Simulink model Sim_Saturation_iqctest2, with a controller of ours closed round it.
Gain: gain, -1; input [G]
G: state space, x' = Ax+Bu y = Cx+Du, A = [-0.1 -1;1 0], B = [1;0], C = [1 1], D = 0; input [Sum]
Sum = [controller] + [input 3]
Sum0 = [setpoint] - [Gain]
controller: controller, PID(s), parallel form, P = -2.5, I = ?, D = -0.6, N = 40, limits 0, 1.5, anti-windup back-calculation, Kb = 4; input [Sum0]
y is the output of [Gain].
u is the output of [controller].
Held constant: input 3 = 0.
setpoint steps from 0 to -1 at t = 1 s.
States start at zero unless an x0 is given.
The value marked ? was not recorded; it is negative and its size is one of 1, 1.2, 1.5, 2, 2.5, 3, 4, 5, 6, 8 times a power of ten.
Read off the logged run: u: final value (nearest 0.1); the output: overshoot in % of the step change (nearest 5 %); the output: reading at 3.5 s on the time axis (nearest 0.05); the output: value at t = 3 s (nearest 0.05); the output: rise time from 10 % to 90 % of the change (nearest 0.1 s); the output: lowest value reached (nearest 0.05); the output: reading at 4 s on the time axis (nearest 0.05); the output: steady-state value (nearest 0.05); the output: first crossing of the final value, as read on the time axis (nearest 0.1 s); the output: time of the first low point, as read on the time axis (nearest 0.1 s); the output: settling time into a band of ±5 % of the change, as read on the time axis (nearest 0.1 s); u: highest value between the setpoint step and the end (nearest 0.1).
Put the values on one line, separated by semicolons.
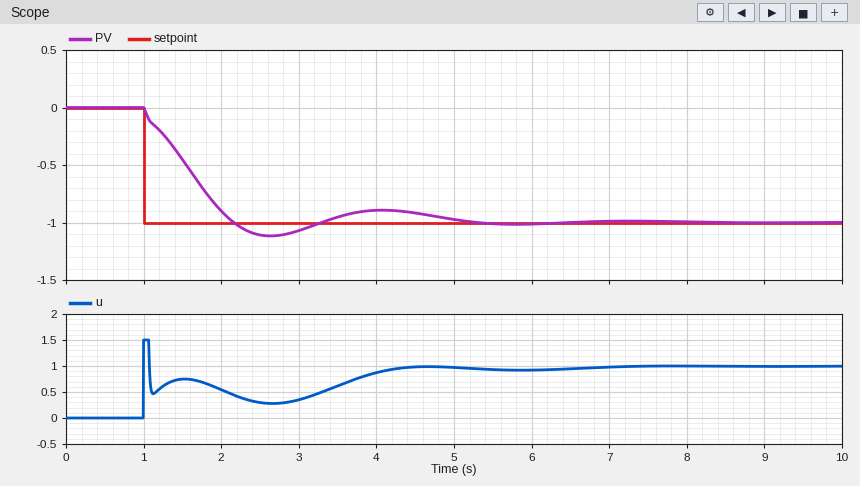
1.0; 10 %; -0.95; -1.05; 0.9 s; -1.10; -0.90; -1.00; 2.2 s; 2.6 s; 4.8 s; 1.5
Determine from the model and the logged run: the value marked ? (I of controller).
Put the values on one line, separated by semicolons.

-5
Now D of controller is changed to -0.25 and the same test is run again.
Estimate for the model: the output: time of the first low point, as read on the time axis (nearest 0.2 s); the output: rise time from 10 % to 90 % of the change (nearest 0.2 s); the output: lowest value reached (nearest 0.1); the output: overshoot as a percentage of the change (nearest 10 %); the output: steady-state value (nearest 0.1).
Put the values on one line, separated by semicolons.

2.2 s; 0.6 s; -1.2; 20 %; -1.0
